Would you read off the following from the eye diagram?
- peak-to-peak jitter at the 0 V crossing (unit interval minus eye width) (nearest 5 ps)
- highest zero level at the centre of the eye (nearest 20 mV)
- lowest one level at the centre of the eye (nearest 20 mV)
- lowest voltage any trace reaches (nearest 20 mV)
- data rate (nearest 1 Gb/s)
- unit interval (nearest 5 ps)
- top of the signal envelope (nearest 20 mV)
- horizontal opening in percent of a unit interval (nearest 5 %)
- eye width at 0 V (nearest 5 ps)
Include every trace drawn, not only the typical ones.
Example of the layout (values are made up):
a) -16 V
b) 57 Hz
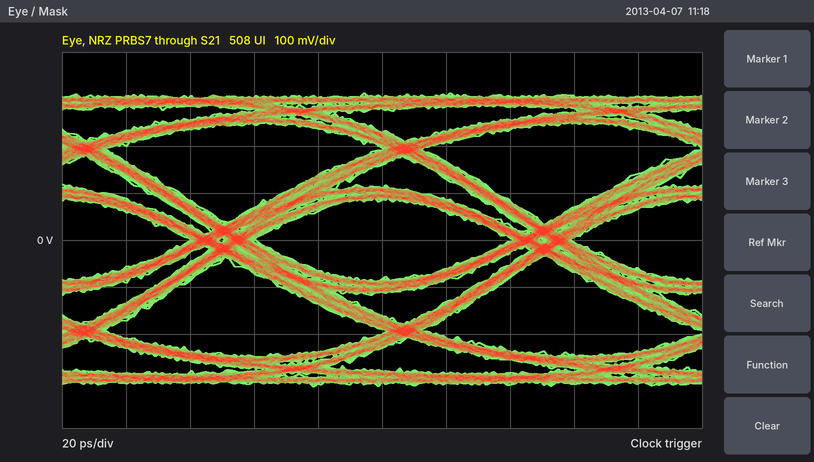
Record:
a) 20 ps
b) -80 mV
c) 80 mV
d) -320 mV
e) 10 Gb/s
f) 100 ps
g) 320 mV
h) 80 %
i) 80 ps
